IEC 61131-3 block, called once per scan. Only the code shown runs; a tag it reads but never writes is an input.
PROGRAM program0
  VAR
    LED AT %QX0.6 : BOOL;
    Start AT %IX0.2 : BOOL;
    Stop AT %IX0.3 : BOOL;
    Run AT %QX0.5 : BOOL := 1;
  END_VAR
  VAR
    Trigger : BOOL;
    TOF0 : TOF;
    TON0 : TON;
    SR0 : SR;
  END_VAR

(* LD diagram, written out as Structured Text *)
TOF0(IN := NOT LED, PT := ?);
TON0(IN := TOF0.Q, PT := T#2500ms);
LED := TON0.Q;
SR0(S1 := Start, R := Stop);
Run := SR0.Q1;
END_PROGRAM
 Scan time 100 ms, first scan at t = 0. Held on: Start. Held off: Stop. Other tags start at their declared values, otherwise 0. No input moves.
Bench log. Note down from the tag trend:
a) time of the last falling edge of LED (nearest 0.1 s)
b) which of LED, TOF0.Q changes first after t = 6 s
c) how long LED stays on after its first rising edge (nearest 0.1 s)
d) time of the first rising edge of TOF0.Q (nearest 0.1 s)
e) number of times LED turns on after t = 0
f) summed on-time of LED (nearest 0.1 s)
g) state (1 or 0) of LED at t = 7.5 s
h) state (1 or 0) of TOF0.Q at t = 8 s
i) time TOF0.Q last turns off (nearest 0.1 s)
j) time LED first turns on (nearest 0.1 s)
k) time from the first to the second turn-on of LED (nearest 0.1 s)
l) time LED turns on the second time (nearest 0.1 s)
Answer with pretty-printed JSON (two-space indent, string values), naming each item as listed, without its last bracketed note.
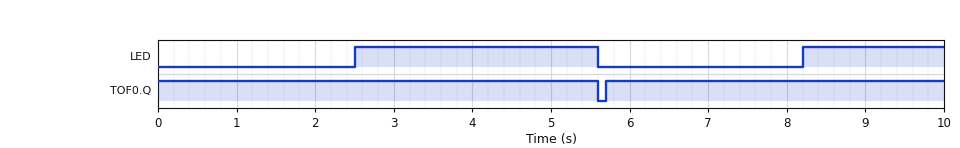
{
  "time of the last falling edge of LED": "5.6 s",
  "which of LED, TOF0.Q changes first after t = 6 s": "LED",
  "how long LED stays on after its first rising edge": "3.1 s",
  "time of the first rising edge of TOF0.Q": "5.7 s",
  "number of times LED turns on after t = 0": "2",
  "summed on-time of LED": "4.9 s",
  "state (1 or 0) of LED at t = 7.5 s": "0",
  "state (1 or 0) of TOF0.Q at t = 8 s": "1",
  "time TOF0.Q last turns off": "5.6 s",
  "time LED first turns on": "2.5 s",
  "time from the first to the second turn-on of LED": "5.7 s",
  "time LED turns on the second time": "8.2 s"
}
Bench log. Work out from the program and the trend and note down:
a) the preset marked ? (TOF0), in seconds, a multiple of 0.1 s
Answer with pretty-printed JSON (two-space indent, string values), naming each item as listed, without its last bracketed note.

{
  "the preset marked ? (TOF0), in seconds, a multiple of 0.1 s": "3.0 s"
}
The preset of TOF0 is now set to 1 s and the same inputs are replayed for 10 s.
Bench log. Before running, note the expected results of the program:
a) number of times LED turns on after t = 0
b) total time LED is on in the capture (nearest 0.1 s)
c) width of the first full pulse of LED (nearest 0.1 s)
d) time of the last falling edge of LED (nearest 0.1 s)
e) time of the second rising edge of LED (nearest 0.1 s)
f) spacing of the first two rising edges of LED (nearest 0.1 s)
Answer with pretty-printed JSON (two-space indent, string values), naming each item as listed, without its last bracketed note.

{
  "number of times LED turns on after t = 0": "3",
  "total time LED is on in the capture": "2.3 s",
  "width of the first full pulse of LED": "1.1 s",
  "time of the last falling edge of LED": "7.3 s",
  "time of the second rising edge of LED": "6.2 s",
  "spacing of the first two rising edges of LED": "3.7 s"
}
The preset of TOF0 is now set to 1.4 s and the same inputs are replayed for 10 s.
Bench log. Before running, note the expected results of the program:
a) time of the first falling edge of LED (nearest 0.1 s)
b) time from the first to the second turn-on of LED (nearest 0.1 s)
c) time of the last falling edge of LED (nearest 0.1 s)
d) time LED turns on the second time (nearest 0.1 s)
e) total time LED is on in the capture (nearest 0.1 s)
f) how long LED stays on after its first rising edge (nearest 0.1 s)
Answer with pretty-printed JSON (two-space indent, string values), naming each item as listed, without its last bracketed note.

{
  "time of the first falling edge of LED": "4.0 s",
  "time from the first to the second turn-on of LED": "4.1 s",
  "time of the last falling edge of LED": "8.1 s",
  "time LED turns on the second time": "6.6 s",
  "total time LED is on in the capture": "3.0 s",
  "how long LED stays on after its first rising edge": "1.5 s"
}
